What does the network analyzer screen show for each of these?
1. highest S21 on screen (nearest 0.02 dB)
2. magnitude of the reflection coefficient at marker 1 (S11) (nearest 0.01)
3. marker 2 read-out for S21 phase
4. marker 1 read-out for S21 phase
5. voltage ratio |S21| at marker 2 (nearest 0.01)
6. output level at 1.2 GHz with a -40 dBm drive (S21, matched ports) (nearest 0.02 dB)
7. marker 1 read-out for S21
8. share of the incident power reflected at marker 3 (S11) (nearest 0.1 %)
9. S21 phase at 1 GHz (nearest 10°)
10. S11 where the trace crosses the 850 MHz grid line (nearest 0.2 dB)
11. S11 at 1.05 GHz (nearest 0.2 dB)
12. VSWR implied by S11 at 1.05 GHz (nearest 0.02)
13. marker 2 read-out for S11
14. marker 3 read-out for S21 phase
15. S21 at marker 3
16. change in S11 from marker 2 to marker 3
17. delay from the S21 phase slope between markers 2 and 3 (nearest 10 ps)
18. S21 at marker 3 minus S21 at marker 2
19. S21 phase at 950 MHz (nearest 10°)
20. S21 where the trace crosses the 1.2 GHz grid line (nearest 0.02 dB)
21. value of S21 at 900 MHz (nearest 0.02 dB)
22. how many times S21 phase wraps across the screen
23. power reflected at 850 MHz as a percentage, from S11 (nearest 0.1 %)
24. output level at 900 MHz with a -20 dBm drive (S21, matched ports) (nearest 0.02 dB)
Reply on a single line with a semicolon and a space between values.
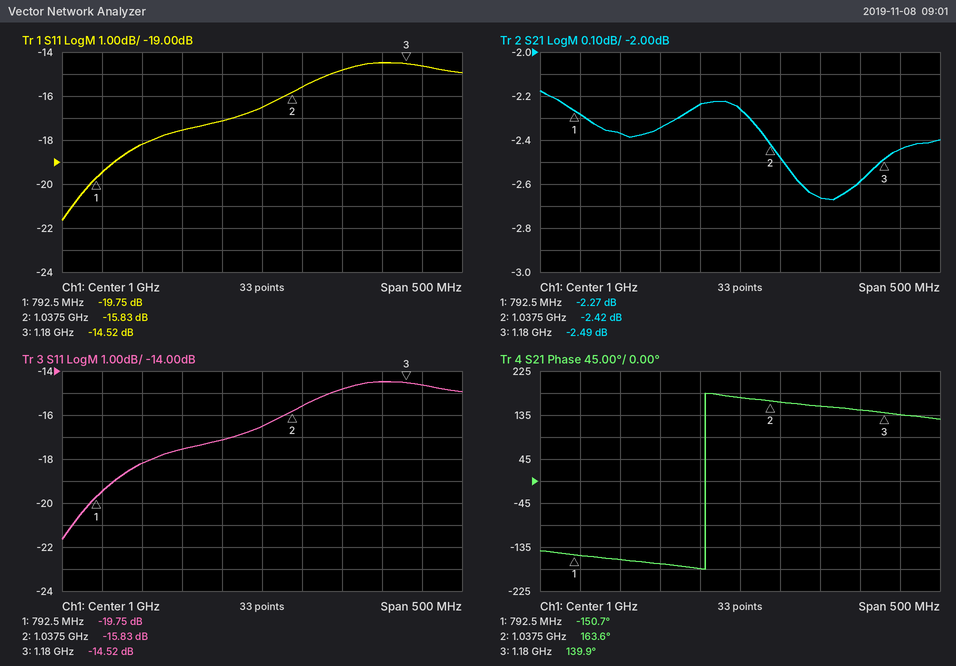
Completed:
-2.18 dB; 0.10; 163.6°; -150.7°; 0.76; -42.44 dBm; -2.27 dB; 3.5 %; 170°; -18.2 dB; -15.6 dB; 1.40; -15.83 dB; 139.9°; -2.49 dB; 1.31 dB; 460 ps; -0.07 dB; -180°; -2.44 dB; -2.34 dB; 1; 1.5 %; -22.34 dBm
